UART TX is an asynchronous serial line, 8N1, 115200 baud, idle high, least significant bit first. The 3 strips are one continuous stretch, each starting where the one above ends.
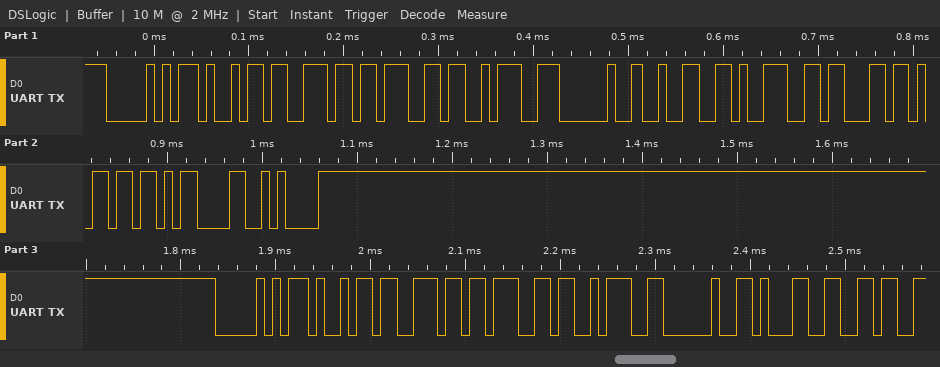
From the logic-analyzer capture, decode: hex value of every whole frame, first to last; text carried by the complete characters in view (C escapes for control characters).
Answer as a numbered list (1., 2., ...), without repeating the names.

1. 50 69 6E 67 3A 20 32 39 63 6D 0D 0A 50 69 6E 67 3A 20 31 36
2. "Ping: 29cm\r\nPing: 16"
